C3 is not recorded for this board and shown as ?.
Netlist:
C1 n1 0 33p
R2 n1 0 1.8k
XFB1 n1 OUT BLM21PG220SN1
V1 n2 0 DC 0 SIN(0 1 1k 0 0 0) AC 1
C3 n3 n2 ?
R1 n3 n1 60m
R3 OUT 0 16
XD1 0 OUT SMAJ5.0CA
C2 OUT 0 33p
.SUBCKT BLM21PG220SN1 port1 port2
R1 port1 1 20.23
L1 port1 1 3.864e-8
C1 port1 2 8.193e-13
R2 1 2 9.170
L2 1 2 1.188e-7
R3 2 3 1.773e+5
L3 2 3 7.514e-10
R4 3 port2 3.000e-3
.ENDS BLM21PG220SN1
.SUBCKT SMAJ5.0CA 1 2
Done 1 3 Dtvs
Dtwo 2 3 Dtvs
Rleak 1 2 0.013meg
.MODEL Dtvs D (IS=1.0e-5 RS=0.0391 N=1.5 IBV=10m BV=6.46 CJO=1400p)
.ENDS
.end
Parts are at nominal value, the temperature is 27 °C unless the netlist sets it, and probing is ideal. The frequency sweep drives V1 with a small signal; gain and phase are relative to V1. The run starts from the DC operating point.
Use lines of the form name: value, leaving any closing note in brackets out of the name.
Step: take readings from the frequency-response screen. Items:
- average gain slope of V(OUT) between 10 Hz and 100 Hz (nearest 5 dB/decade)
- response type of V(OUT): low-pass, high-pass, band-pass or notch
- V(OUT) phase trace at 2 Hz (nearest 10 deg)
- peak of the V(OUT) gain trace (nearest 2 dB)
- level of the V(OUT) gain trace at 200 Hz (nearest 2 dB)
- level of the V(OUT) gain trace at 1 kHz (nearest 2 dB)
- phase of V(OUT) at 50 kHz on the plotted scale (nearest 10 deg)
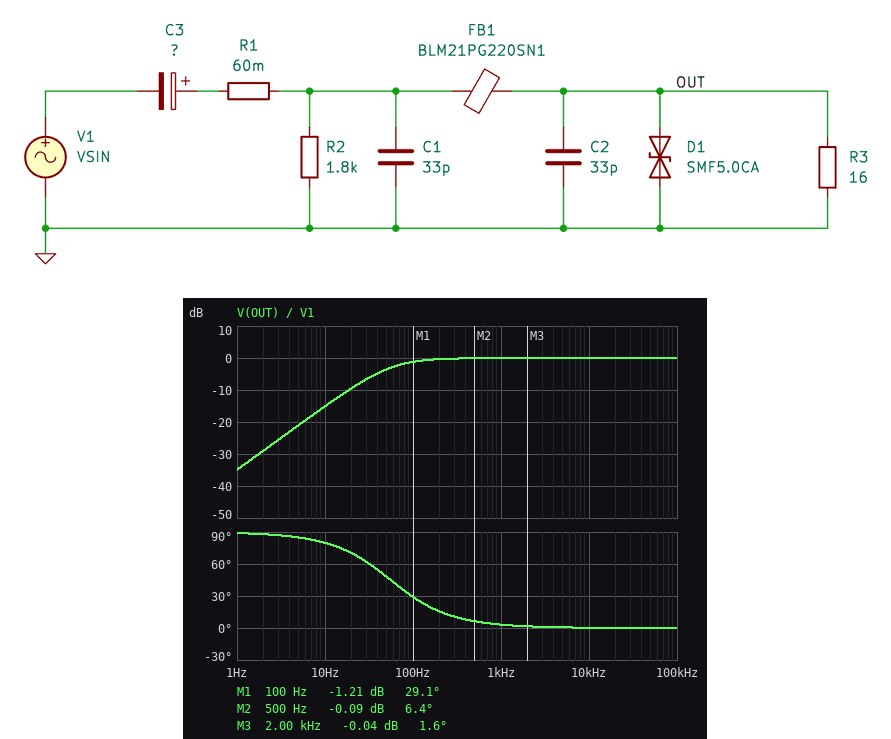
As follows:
average gain slope of V(OUT) between 10 Hz and 100 Hz: 15 dB/decade
response type of V(OUT): low-pass, high-pass, band-pass or notch: high-pass
V(OUT) phase trace at 2 Hz: 90 deg
peak of the V(OUT) gain trace: 0 dB
level of the V(OUT) gain trace at 200 Hz: 0 dB
level of the V(OUT) gain trace at 1 kHz: 0 dB
phase of V(OUT) at 50 kHz on the plotted scale: 0 deg
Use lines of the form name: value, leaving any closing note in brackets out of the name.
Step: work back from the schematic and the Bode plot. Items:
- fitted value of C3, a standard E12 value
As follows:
fitted value of C3, a standard E12 value: 180 µF
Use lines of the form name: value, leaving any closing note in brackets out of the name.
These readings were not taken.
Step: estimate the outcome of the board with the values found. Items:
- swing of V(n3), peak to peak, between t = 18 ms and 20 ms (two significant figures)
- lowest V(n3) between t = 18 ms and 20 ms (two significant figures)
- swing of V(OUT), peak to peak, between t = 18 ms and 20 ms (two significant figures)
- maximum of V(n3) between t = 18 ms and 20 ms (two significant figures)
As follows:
swing of V(n3), peak to peak, between t = 18 ms and 20 ms: 2.0 V
lowest V(n3) between t = 18 ms and 20 ms: -1.0 V
swing of V(OUT), peak to peak, between t = 18 ms and 20 ms: 2.0 V
maximum of V(n3) between t = 18 ms and 20 ms: 1.0 V
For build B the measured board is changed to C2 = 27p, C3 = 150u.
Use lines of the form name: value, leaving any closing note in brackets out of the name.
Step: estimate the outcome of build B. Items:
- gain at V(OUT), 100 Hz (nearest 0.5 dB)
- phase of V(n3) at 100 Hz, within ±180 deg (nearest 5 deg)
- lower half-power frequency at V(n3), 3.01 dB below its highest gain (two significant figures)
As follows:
gain at V(OUT), 100 Hz: -1.5 dB
phase of V(n3) at 100 Hz, within ±180 deg: 35 deg
lower half-power frequency at V(n3), 3.01 dB below its highest gain: 67 Hz
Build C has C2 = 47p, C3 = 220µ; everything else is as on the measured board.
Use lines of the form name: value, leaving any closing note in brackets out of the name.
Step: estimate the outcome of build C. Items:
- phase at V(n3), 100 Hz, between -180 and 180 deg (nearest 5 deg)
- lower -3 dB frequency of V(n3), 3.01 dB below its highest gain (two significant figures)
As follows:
phase at V(n3), 100 Hz, between -180 and 180 deg: 25 deg
lower -3 dB frequency of V(n3), 3.01 dB below its highest gain: 46 Hz
